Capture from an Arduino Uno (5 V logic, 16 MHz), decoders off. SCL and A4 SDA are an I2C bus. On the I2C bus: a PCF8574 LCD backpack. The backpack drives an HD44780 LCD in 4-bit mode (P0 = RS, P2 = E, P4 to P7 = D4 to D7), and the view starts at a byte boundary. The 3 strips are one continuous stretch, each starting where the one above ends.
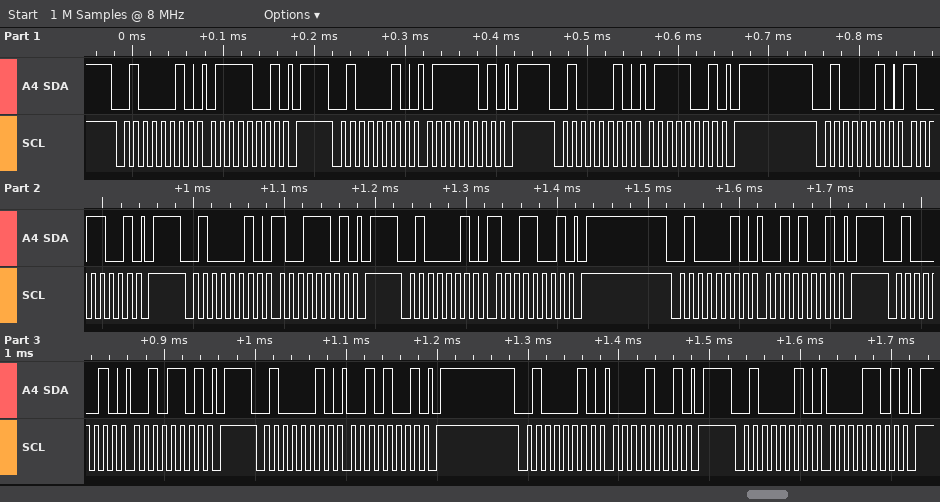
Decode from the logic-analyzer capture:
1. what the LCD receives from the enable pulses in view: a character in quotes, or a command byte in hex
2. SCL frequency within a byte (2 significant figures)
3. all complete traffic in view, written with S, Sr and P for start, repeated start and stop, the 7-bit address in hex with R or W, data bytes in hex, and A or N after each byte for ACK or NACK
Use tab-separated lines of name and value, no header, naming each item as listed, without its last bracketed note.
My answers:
what the LCD receives from the enable pulses in view: a character in quotes, or a command byte in hex	'y'
SCL frequency within a byte	100 kHz
all complete traffic in view, written with S, Sr and P for start, repeated start and stop, the 7-bit address in hex with R or W, data bytes in hex, and A or N after each byte for ACK or NACK	S 21W A 79 A P S 21W A 7D A P S 21W A 79 A P S 21W A 99 A P S 21W A 9D A P S 21W A 99 A P S 21W A 29 A P S 21W A 2D A P S 21W A 29 A P S 21W A 09 A P S 21W A 0D A P
